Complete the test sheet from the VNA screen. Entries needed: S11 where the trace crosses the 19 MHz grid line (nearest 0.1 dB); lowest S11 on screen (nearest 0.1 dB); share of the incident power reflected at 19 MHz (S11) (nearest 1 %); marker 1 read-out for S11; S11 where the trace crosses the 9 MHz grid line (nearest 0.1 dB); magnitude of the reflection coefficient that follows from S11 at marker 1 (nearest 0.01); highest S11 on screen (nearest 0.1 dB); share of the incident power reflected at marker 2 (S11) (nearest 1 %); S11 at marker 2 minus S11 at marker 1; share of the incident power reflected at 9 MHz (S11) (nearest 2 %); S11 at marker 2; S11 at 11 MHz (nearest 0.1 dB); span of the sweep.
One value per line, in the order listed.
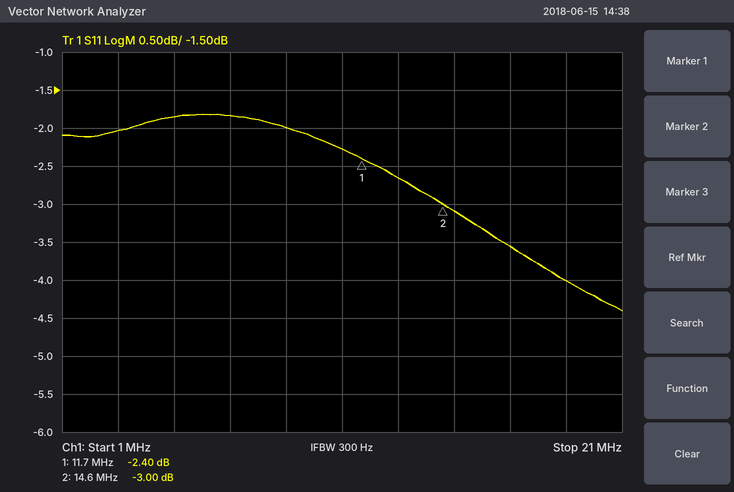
-4.0 dB
-4.4 dB
40 %
-2.40 dB
-2.0 dB
0.76
-1.8 dB
50 %
-0.60 dB
64 %
-3.00 dB
-2.3 dB
20 MHz
